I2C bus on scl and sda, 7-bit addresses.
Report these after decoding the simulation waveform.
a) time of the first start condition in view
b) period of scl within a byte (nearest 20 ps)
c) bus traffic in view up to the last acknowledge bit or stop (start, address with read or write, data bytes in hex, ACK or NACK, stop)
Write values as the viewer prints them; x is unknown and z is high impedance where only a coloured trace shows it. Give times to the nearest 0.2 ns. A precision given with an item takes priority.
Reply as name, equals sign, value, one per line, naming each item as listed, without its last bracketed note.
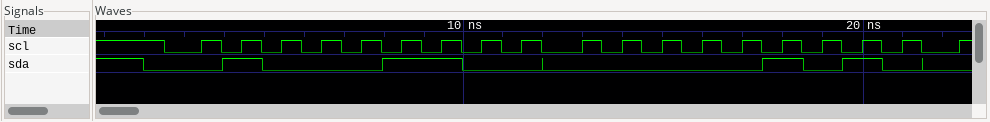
time of the first start condition in view = 2 ns
period of scl within a byte = 1000 ps
bus traffic in view up to the last acknowledge bit or stop = start, address 23 write ACK, 05 ACK
